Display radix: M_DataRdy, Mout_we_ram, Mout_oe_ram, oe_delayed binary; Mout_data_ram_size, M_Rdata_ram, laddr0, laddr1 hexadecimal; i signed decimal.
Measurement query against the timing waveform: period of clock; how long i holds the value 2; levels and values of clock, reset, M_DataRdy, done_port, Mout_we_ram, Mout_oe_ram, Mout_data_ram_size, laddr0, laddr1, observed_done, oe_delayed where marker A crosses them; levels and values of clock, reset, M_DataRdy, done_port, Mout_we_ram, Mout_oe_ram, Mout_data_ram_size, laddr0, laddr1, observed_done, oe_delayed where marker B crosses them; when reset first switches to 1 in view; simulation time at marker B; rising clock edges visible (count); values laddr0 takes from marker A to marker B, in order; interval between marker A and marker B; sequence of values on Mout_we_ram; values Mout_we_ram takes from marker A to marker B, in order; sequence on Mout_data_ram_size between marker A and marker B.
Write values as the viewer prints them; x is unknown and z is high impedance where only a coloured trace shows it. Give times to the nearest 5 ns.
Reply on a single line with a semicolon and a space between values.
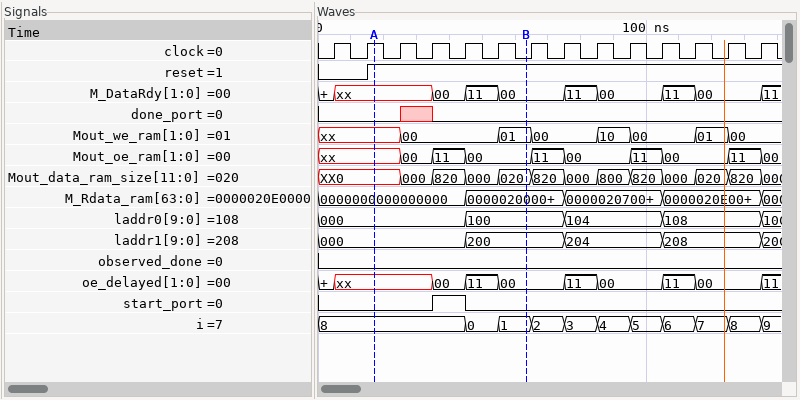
10 ns; 10 ns; clock=1, reset=1, M_DataRdy=xx, done_port=0, Mout_we_ram=xx, Mout_oe_ram=xx, Mout_data_ram_size=XX0, laddr0=000, laddr1=000, observed_done=0, oe_delayed=xx; clock=0, reset=1, M_DataRdy=00, done_port=0, Mout_we_ram=01, Mout_oe_ram=00, Mout_data_ram_size=020, laddr0=100, laddr1=200, observed_done=0, oe_delayed=00; 15 ns; 65 ns; 14; 000, 100; 45 ns; xx, 00, 01, 00, 10, 00, 01, 00; xx, 00, 01; XX0, 000, 820, 000, 020
